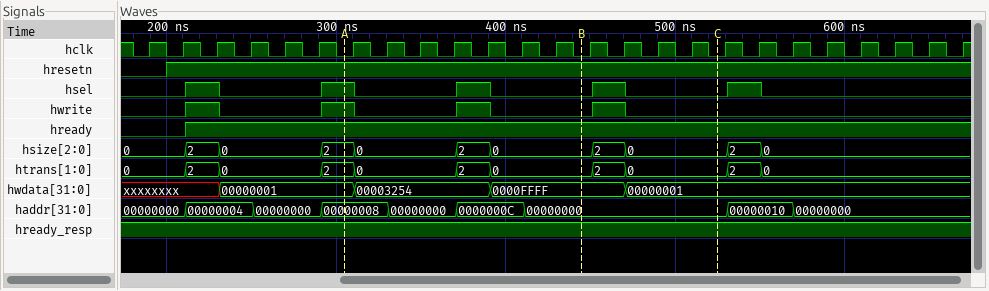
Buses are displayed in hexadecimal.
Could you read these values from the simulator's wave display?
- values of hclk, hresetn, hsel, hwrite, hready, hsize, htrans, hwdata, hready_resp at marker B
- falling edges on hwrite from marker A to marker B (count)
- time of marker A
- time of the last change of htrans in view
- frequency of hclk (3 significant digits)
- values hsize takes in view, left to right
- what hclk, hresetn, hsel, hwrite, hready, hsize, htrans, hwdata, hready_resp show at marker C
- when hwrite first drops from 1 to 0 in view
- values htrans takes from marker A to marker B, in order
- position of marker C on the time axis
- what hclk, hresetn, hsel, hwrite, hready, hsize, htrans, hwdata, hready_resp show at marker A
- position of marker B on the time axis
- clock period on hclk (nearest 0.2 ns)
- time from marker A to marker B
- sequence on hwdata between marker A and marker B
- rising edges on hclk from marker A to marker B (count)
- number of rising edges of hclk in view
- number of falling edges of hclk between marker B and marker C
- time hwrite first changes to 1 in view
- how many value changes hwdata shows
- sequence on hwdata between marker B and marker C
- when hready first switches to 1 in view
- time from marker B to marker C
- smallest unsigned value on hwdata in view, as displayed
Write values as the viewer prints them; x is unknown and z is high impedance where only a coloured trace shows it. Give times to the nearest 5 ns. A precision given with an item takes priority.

hclk=0, hresetn=1, hsel=0, hwrite=0, hready=1, hsize=0, htrans=0, hwdata=0000FFFF, hready_resp=1
2
305 ns
550 ns
50.0 MHz
0, 2, 0, 2, 0, 2, 0, 2, 0, 2, 0
hclk=0, hresetn=1, hsel=0, hwrite=0, hready=1, hsize=0, htrans=0, hwdata=00000001, hready_resp=1
230 ns
2, 0, 2, 0
525 ns
hclk=0, hresetn=1, hsel=1, hwrite=1, hready=1, hsize=2, htrans=2, hwdata=00000001, hready_resp=1
445 ns
20 ns
140 ns
00000001, 00003254, 0000FFFF
7
25
4
210 ns
4
0000FFFF, 00000001
210 ns
80 ns
00000001
